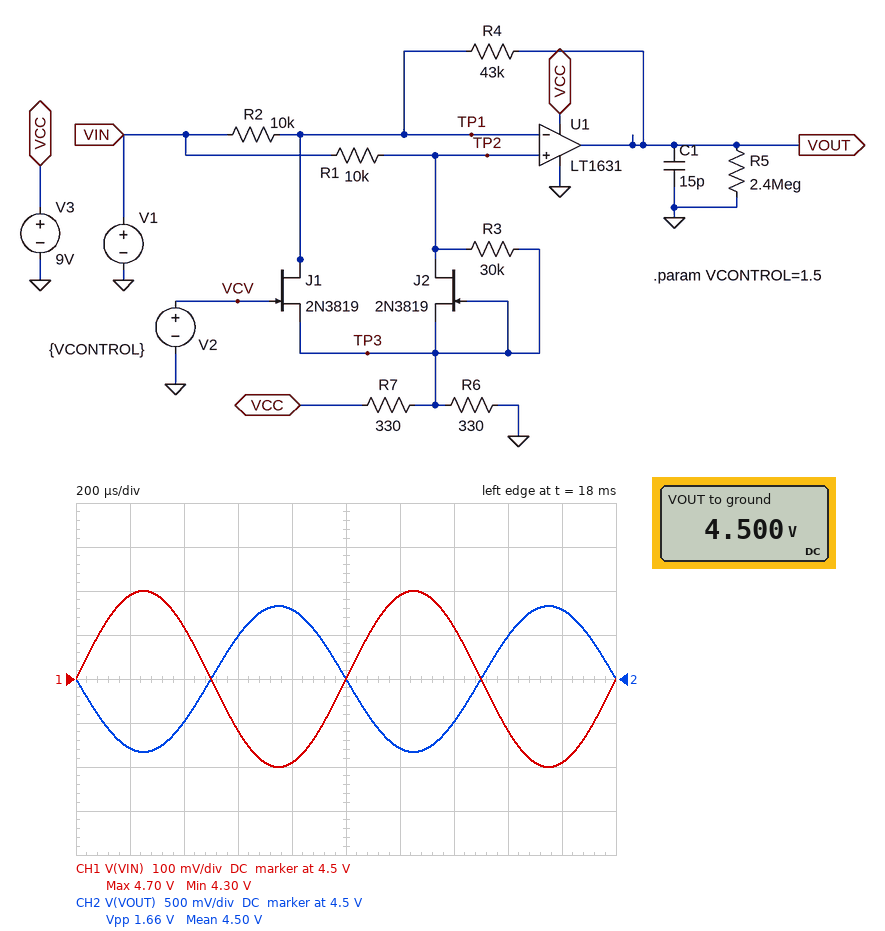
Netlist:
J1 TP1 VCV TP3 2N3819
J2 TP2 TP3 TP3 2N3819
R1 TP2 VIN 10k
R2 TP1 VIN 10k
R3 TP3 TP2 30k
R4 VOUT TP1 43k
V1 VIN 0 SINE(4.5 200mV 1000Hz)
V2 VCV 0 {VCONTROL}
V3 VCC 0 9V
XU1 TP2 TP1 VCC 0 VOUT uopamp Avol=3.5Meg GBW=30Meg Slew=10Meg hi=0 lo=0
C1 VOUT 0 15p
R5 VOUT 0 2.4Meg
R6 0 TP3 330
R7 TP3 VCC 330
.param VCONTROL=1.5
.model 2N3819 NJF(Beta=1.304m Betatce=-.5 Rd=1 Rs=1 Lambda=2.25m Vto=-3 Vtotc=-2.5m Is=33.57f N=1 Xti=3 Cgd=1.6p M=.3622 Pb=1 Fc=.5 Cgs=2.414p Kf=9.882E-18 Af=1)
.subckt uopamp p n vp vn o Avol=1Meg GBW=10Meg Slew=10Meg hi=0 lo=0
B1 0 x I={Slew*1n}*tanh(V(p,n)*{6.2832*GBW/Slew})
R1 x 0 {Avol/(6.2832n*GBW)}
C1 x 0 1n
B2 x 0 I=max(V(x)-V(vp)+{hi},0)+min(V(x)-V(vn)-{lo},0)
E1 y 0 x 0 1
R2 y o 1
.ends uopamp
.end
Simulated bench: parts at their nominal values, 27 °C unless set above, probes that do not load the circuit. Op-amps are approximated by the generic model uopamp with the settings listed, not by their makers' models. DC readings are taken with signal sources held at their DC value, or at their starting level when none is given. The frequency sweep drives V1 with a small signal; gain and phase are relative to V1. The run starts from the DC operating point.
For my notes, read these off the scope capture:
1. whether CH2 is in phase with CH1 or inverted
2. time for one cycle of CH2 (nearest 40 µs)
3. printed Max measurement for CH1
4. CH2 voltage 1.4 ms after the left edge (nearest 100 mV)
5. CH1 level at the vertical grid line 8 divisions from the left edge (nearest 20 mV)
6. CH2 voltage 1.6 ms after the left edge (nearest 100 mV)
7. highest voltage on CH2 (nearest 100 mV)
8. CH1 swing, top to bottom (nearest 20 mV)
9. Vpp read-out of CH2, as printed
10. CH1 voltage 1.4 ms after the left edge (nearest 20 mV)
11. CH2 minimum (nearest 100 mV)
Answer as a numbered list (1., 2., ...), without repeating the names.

1. inverted
2. 1.00 ms
3. 4.70 V
4. 4.0 V
5. 4.38 V
6. 5.0 V
7. 5.3 V
8. 400 mV
9. 1.66 V
10. 4.62 V
11. 3.7 V
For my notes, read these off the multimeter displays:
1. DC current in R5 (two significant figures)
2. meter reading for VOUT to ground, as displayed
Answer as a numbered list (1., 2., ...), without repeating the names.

1. 1.9 µA
2. 4.500 V
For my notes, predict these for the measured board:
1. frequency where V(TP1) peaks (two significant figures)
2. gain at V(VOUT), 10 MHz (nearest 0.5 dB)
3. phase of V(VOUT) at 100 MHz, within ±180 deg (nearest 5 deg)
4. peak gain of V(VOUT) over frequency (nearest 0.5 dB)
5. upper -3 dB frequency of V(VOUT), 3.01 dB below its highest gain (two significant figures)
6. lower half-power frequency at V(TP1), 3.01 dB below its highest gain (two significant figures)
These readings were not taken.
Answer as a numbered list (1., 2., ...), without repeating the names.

1. 12 MHz
2. 7.5 dB
3. 5 deg
4. 12.5 dB
5. 7.2 MHz
6. 4.7 MHz
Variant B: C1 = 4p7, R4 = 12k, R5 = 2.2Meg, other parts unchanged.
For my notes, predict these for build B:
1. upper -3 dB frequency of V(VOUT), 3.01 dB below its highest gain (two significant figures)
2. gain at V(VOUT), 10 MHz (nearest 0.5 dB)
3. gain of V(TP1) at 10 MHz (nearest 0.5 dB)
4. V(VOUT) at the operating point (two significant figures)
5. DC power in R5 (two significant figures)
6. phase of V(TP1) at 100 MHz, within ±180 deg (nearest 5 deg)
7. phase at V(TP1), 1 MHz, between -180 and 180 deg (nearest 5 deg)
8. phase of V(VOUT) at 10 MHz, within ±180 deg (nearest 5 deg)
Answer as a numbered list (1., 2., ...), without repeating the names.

1. 19 MHz
2. 0.5 dB
3. -8.5 dB
4. 4.5 V
5. 9.2 µW
6. -70 deg
7. 50 deg
8. 135 deg
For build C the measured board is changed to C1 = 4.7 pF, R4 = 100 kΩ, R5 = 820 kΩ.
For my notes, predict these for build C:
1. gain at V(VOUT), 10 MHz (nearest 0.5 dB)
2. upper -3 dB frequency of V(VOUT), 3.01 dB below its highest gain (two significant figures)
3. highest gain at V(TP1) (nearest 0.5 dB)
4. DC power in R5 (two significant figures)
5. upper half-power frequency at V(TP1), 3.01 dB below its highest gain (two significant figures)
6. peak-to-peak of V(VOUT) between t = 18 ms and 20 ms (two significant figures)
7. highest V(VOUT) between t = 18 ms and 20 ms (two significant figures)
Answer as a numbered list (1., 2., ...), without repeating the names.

1. 8.5 dB
2. 3.1 MHz
3. -1.0 dB
4. 25 µW
5. 24 MHz
6. 3.9 V
7. 6.4 V
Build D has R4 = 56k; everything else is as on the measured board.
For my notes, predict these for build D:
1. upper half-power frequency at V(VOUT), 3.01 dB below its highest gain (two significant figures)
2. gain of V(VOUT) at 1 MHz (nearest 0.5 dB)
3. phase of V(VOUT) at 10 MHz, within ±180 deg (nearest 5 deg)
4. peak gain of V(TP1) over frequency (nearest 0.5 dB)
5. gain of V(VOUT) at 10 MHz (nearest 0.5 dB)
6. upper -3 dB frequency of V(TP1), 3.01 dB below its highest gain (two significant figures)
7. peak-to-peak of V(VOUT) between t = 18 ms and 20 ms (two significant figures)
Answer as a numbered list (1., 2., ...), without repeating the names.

1. 5.6 MHz
2. 14.5 dB
3. 90 deg
4. -1.5 dB
5. 8.0 dB
6. 27 MHz
7. 2.2 V
